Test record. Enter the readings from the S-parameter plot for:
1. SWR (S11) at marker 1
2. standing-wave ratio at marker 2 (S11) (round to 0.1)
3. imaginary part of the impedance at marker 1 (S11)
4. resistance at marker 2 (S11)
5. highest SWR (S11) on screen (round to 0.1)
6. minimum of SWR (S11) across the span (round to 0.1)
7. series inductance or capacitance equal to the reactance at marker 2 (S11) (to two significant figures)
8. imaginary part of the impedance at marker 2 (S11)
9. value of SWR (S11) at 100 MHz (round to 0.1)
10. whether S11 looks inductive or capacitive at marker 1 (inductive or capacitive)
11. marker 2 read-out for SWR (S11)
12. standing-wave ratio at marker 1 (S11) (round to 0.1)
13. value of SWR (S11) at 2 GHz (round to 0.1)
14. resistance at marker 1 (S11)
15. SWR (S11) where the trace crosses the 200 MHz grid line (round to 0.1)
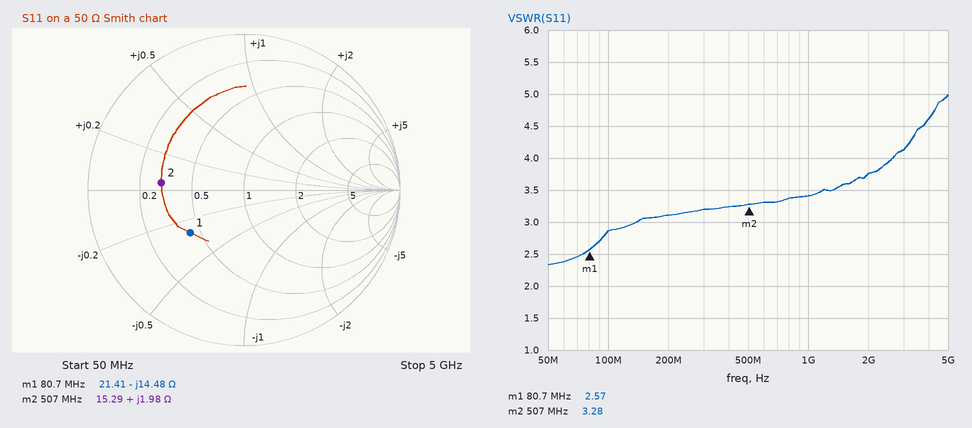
2.57
3.3
-14.48 Ω
15.29 Ω
5.0
2.3
620 pH
+1.98 Ω
2.9
capacitive
3.28
2.6
3.8
21.41 Ω
3.1
